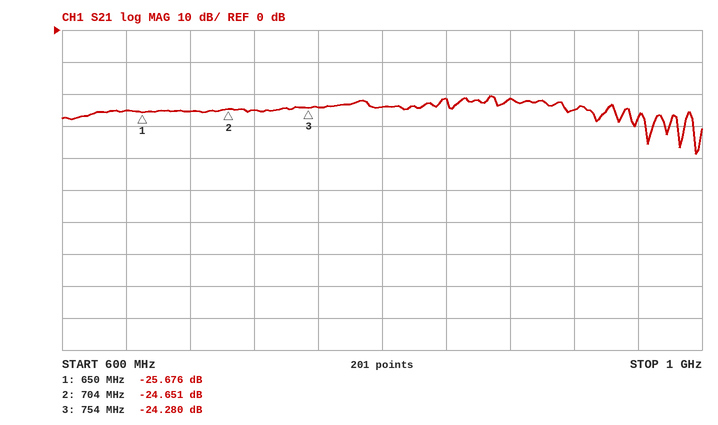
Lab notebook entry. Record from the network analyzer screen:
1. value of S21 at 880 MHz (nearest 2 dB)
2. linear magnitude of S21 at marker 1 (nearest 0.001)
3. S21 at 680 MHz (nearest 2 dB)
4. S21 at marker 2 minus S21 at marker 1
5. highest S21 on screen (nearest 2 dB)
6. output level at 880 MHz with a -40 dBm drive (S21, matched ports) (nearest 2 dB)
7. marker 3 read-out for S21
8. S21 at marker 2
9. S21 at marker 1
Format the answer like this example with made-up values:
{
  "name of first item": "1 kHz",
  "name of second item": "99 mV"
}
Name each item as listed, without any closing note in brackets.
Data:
{
  "value of S21 at 880 MHz": "-22 dB",
  "linear magnitude of S21 at marker 1": "0.052",
  "S21 at 680 MHz": "-26 dB",
  "S21 at marker 2 minus S21 at marker 1": "1.025 dB",
  "highest S21 on screen": "-20 dB",
  "output level at 880 MHz with a -40 dBm drive (S21, matched ports)": "-62 dBm",
  "marker 3 read-out for S21": "-24.280 dB",
  "S21 at marker 2": "-24.651 dB",
  "S21 at marker 1": "-25.676 dB"
}
